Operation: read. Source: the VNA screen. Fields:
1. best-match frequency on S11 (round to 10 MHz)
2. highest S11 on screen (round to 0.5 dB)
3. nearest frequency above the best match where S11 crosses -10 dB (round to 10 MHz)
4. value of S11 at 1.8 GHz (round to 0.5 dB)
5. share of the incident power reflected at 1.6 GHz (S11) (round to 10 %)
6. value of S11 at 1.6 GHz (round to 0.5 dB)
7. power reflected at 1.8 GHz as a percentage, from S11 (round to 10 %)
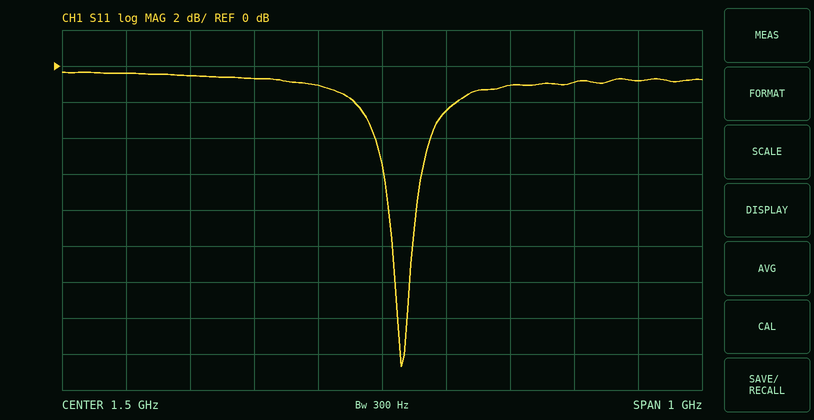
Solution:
1.53 GHz
-0.5 dB
1.55 GHz
-1.0 dB
60 %
-2.5 dB
80 %
